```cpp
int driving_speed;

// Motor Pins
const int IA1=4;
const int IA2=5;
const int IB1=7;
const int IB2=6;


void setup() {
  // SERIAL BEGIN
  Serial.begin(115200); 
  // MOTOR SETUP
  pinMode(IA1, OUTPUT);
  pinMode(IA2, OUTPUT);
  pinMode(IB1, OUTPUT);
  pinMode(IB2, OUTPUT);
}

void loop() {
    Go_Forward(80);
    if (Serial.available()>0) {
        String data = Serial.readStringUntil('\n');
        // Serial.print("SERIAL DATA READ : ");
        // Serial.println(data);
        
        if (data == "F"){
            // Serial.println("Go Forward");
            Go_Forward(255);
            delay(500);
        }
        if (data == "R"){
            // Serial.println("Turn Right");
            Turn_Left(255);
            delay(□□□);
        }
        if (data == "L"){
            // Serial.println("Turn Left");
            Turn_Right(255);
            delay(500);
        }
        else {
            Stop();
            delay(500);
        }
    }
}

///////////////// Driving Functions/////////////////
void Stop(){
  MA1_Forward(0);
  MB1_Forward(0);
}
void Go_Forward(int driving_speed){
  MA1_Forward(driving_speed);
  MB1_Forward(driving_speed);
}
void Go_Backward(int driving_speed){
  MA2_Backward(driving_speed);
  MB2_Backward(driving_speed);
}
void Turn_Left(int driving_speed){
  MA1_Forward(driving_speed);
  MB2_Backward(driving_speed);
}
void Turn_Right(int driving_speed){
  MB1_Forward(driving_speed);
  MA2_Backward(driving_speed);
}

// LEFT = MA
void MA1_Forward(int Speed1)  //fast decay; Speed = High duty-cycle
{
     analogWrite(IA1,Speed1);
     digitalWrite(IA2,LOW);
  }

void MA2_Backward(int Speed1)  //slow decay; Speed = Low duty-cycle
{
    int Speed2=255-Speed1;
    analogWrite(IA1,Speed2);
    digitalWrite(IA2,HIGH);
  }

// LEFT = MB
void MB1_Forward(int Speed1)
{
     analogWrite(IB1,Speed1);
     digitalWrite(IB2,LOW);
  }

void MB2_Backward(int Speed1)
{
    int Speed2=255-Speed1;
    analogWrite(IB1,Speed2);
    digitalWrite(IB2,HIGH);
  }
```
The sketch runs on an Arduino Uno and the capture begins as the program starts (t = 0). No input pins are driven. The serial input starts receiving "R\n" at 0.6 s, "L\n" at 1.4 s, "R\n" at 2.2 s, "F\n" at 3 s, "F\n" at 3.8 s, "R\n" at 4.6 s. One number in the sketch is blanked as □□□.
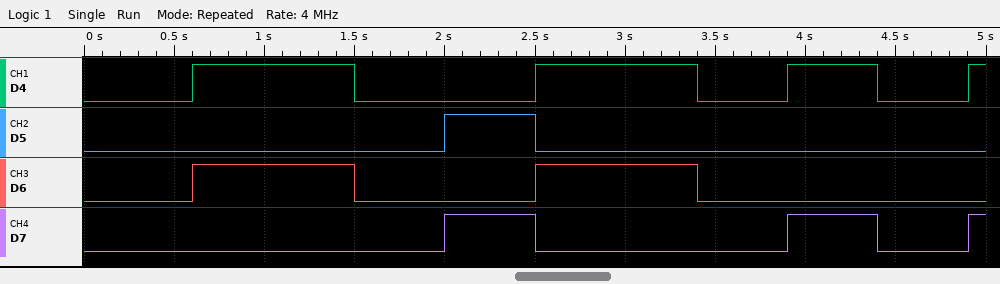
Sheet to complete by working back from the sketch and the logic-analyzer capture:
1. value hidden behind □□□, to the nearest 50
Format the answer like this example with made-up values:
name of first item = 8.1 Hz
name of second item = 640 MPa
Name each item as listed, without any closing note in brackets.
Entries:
value hidden behind □□□, to the nearest 50 = 900
